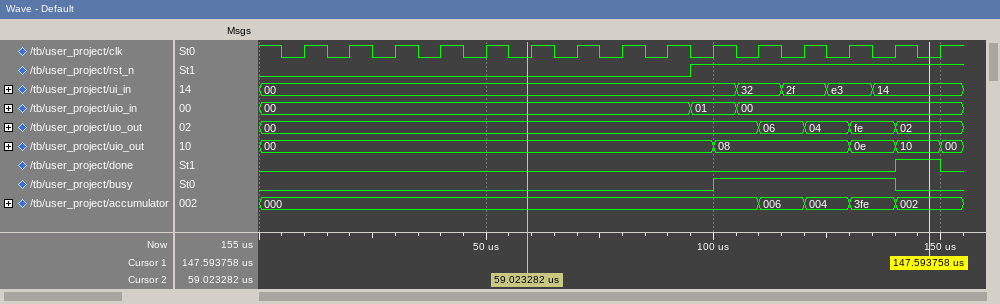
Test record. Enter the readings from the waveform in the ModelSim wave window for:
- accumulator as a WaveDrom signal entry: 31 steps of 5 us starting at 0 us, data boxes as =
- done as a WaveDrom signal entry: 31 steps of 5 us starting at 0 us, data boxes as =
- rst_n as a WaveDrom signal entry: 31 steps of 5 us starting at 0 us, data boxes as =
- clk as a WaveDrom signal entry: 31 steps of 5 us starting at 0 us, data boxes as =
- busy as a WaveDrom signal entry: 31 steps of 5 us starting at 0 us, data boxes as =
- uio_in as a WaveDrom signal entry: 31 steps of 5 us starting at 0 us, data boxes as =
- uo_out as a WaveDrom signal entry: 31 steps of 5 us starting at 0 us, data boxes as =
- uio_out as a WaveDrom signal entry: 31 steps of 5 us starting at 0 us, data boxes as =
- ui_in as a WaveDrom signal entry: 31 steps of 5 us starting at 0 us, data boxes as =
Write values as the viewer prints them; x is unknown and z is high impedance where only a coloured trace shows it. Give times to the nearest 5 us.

{name: 'accumulator', wave: '=.....................=.=.=.=..', data: '000 006 004 3fe 002'}
{name: 'done', wave: '0...........................1.0'}
{name: 'rst_n', wave: '0..................1...........'}
{name: 'clk', wave: '1010101010101010101010101010101'}
{name: 'busy', wave: '0...................1.......0..'}
{name: 'uio_in', wave: '=..................=.=.........', data: '00 01 00'}
{name: 'uo_out', wave: '=.....................=.=.=.=..', data: '00 06 04 fe 02'}
{name: 'uio_out', wave: '=...................=.....=.=.=', data: '00 08 0e 10 00'}
{name: 'ui_in', wave: '=....................=.=.=.=...', data: '00 32 2f e3 14'}
